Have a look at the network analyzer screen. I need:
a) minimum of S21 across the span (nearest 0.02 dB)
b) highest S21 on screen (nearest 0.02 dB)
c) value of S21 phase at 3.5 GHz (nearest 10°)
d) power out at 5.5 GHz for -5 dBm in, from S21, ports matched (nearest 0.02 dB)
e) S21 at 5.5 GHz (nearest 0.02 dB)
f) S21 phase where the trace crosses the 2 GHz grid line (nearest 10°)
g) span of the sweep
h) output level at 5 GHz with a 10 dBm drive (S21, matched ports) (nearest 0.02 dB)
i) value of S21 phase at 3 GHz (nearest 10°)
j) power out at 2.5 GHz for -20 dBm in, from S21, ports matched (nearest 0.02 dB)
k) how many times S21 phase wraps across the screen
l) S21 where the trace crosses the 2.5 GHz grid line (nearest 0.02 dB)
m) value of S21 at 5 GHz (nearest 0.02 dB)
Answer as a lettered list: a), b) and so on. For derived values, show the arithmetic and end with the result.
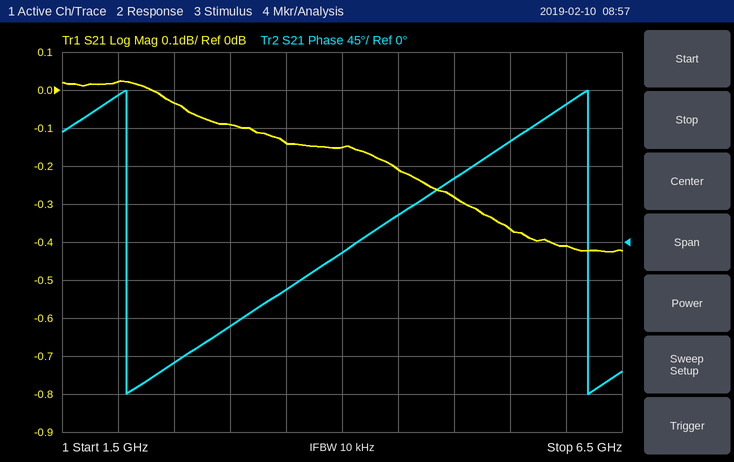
a) -0.42 dB
b) 0.02 dB
c) -60°
d) -5 dBm + (-0.36 dB) = -5.36 dBm
e) -0.36 dB
f) 170°
g) 5 GHz
h) 10 dBm + (-0.28 dB) = 9.72 dBm
i) -100°
j) -20 dBm + (-0.04 dB) = -20.04 dBm
k) 2
l) -0.04 dB
m) -0.28 dB
